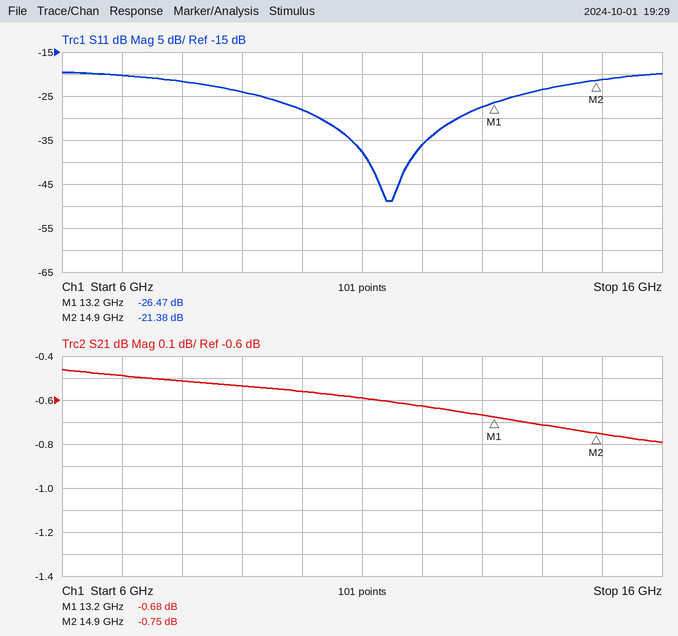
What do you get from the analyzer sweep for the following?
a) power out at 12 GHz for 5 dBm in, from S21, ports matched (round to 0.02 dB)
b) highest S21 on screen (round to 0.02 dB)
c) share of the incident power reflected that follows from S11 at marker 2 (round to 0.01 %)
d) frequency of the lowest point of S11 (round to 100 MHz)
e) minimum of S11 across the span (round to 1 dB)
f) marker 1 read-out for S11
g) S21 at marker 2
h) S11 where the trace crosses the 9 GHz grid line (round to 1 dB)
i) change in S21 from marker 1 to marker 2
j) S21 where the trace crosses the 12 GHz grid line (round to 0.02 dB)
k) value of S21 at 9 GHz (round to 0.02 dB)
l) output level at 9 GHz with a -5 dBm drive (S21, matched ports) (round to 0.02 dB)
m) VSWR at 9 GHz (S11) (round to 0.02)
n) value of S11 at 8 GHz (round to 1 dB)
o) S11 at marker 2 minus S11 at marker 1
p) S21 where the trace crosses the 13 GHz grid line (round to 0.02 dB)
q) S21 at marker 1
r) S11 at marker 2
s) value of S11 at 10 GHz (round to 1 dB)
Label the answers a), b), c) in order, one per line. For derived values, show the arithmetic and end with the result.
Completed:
a) 5 dBm + (-0.62 dB) = 4.38 dBm
b) -0.46 dB
c) 10^(-21.38/10) ≈ 0.73 %
d) 11.4 GHz
e) -49 dB
f) -26.47 dB
g) -0.75 dB
h) -24 dB
i) -0.75 − (-0.68) = -0.07 dB
j) -0.62 dB
k) -0.54 dB
l) -5 dBm + (-0.54 dB) = -5.54 dBm
m) |Γ| = 10^(-24/20) = 0.0631; VSWR = (1 + 0.0631)/(1 − 0.0631) ≈ 1.13, so 1.14 to the nearest 0.02
n) -22 dB
o) -21.38 − (-26.47) = 5.09 dB
p) -0.66 dB
q) -0.68 dB
r) -21.38 dB
s) -28 dB
